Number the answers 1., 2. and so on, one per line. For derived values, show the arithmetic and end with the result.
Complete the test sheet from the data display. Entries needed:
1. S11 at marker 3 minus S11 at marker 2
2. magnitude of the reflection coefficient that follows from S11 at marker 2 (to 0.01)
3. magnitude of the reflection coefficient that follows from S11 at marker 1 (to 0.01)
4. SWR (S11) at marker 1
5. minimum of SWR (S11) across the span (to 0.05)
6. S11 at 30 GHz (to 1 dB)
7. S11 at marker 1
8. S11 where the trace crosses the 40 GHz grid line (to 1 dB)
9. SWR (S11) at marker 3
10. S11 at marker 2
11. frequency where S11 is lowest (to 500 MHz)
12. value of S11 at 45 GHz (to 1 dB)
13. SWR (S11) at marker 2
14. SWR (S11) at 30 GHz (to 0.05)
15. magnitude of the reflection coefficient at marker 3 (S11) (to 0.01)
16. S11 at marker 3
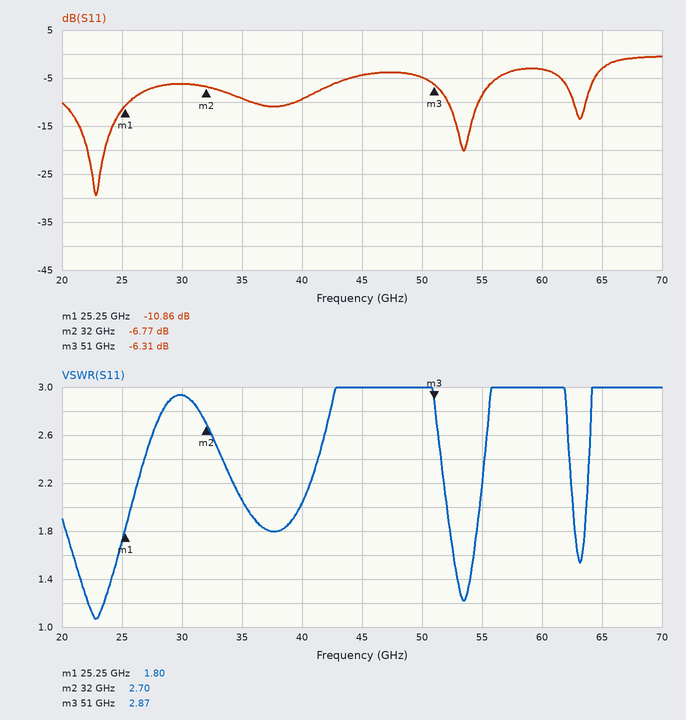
1. -6.31 − (-6.77) = 0.46 dB
2. 10^(-6.77/20) ≈ 0.46
3. 10^(-10.86/20) ≈ 0.29
4. 1.80
5. 1.05
6. -6 dB
7. -10.86 dB
8. -9 dB
9. 2.87
10. -6.77 dB
11. 23.0 GHz
12. -4 dB
13. 2.70
14. 2.95
15. 10^(-6.31/20) ≈ 0.48
16. -6.31 dB
